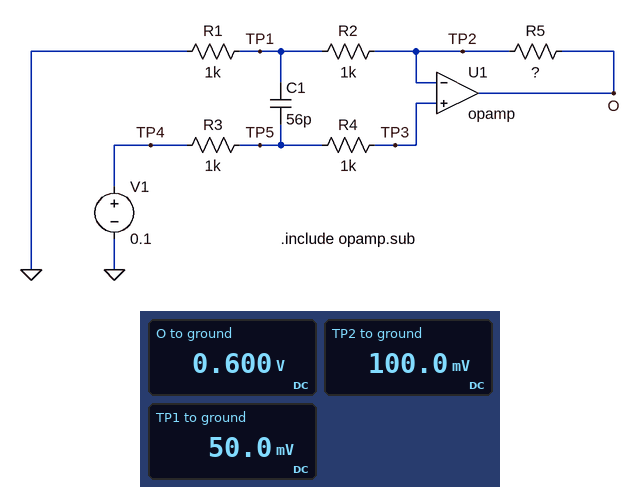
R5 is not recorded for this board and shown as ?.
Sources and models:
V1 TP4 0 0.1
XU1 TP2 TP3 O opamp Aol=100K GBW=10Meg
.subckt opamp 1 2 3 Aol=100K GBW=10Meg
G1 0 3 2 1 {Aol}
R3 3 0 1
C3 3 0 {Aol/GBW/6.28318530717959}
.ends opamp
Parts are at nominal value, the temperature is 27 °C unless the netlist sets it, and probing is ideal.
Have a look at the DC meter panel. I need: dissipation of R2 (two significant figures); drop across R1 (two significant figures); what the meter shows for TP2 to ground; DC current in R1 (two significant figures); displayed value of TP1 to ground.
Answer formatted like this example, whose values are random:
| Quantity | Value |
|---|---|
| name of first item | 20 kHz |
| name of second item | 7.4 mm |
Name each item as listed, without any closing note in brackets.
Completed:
| Quantity | Value |
|---|---|
| dissipation of R2 | 2.5 µW |
| drop across R1 | 50 mV |
| what the meter shows for TP2 to ground | 100.0 mV |
| DC current in R1 | 50 µA |
| displayed value of TP1 to ground | 50.0 mV |
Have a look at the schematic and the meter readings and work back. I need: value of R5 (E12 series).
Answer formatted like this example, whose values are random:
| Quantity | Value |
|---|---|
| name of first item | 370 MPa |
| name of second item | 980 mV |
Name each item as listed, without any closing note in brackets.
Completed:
| Quantity | Value |
|---|---|
| value of R5 | 10 kΩ |
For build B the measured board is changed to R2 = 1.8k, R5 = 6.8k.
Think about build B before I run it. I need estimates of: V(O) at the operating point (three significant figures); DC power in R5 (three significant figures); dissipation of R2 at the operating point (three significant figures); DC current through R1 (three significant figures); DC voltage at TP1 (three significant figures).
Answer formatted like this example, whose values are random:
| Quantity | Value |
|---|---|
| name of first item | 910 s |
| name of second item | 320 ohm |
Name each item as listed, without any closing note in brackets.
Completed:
| Quantity | Value |
|---|---|
| V(O) at the operating point | 343 mV |
| DC power in R5 | 8.67 µW |
| dissipation of R2 at the operating point | 2.30 µW |
| DC current through R1 | 35.7 µA |
| DC voltage at TP1 | 35.7 mV |
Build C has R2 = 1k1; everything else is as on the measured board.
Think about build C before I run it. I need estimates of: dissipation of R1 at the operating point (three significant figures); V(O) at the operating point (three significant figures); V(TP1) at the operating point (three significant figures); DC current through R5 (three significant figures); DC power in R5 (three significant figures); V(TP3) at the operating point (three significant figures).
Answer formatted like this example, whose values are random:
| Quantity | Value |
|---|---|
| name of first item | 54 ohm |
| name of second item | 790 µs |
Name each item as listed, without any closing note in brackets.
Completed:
| Quantity | Value |
|---|---|
| dissipation of R1 at the operating point | 2.27 µW |
| V(O) at the operating point | 576 mV |
| V(TP1) at the operating point | 47.6 mV |
| DC current through R5 | 47.6 µA |
| DC power in R5 | 22.7 µW |
| V(TP3) at the operating point | 100 mV |
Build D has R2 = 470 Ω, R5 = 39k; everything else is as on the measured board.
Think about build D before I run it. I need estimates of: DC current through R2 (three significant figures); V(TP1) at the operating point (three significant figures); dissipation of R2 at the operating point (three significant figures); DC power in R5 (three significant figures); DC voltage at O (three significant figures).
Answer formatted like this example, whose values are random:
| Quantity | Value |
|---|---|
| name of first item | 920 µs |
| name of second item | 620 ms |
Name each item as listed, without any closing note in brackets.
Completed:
| Quantity | Value |
|---|---|
| DC current through R2 | 68.0 µA |
| V(TP1) at the operating point | 68.0 mV |
| dissipation of R2 at the operating point | 2.17 µW |
| DC power in R5 | 180 µW |
| DC voltage at O | 2.75 V |
